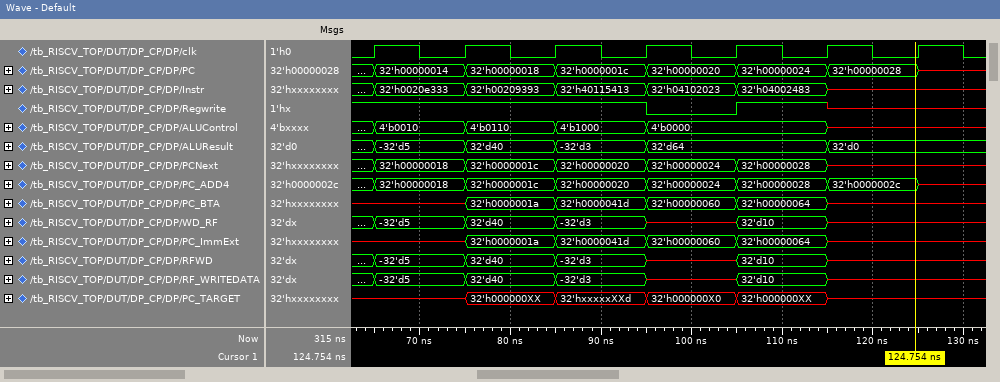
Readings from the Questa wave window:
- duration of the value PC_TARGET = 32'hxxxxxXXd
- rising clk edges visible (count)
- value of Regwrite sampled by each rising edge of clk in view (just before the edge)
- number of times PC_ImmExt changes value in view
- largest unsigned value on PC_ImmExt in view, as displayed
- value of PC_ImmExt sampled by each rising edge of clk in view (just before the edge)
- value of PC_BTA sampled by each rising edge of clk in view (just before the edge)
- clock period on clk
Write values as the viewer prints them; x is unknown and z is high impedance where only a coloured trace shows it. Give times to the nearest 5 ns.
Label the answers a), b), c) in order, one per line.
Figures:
a) 10 ns
b) 7
c) 1 1 1 1 0 1 x
d) 5
e) 32'h0000041d
f) x, x, 32'h0000001a, 32'h0000041d, 32'h00000060, 32'h00000064, x
g) x, x, 32'h0000001a, 32'h0000041d, 32'h00000060, 32'h00000064, x
h) 10 ns
